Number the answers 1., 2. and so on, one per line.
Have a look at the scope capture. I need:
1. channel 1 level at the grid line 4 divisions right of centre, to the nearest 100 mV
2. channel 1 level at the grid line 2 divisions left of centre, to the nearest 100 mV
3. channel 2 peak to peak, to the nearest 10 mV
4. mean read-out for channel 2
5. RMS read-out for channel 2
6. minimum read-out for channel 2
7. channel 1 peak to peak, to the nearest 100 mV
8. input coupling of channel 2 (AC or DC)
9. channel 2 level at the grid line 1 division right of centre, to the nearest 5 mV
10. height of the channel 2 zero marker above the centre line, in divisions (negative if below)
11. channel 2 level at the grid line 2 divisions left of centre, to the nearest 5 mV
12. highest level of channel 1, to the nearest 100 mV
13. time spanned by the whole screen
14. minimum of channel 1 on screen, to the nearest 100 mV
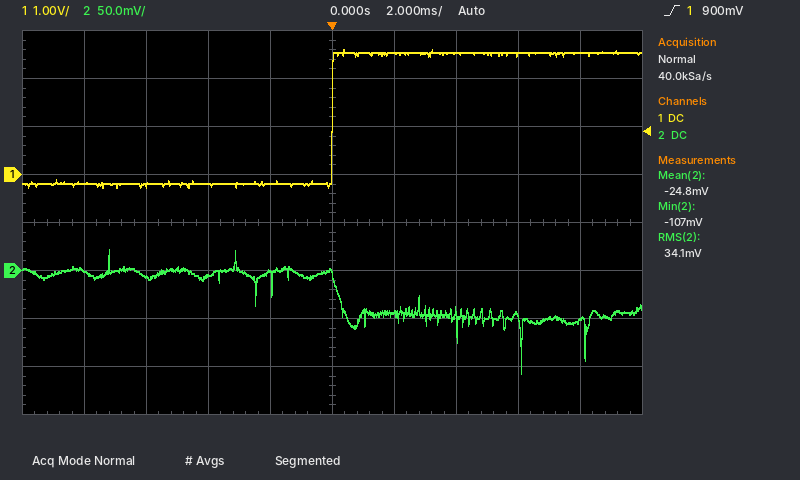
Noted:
1. 2.5 V
2. -200 mV
3. 130 mV
4. -24.8 mV
5. 34.1 mV
6. -107 mV
7. 2.9 V
8. DC
9. -45 mV
10. -1.0 div
11. -5 mV
12. 2.6 V
13. 20 ms
14. -300 mV
